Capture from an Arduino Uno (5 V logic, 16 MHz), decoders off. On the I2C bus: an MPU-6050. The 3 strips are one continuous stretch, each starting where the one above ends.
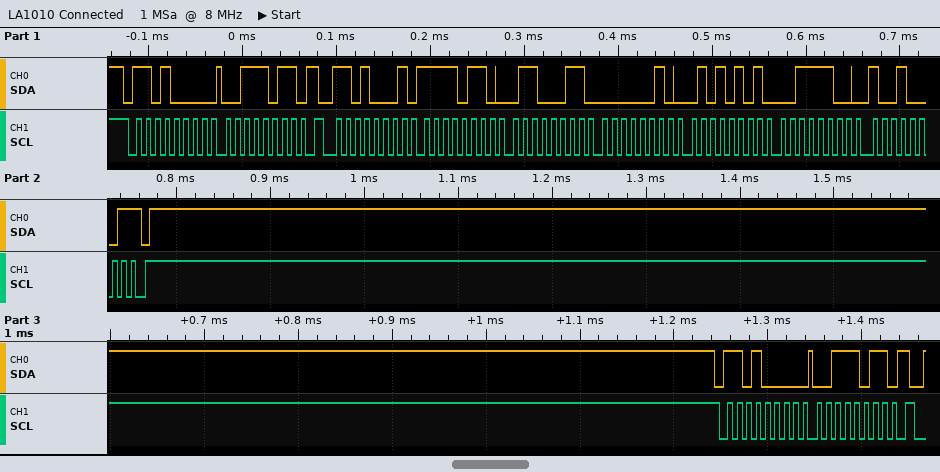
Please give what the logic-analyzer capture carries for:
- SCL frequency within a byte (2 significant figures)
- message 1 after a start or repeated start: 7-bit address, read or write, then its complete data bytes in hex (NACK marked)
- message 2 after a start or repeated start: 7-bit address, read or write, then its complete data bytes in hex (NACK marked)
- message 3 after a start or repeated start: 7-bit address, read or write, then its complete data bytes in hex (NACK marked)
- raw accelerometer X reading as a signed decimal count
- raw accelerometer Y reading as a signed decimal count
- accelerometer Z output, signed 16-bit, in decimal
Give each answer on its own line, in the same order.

100 kHz
0x68 write: 3B
0x68 read: F6 63 02 55 3C 91 NACK
0x68 write: 3B
-2461
597
15505
